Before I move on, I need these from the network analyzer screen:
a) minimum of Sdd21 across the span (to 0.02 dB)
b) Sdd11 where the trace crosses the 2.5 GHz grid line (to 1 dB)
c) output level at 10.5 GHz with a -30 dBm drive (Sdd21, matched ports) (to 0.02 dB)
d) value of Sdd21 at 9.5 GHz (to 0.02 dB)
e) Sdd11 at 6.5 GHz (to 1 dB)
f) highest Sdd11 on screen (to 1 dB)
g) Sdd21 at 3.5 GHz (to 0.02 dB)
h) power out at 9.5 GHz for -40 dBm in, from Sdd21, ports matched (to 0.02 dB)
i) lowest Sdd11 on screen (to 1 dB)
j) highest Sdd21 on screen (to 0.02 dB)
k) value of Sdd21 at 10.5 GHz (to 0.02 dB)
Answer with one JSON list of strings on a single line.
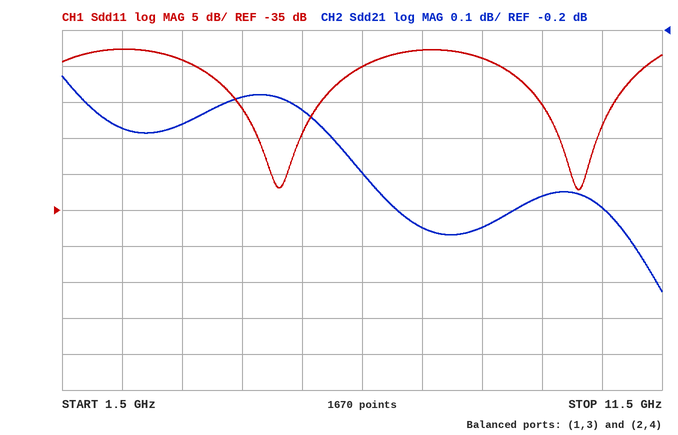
["-0.92 dB", "-13 dB", "-30.70 dBm", "-0.66 dB", "-15 dB", "-13 dB", "-0.46 dB", "-40.66 dBm", "-32 dB", "-0.32 dB", "-0.70 dB"]
